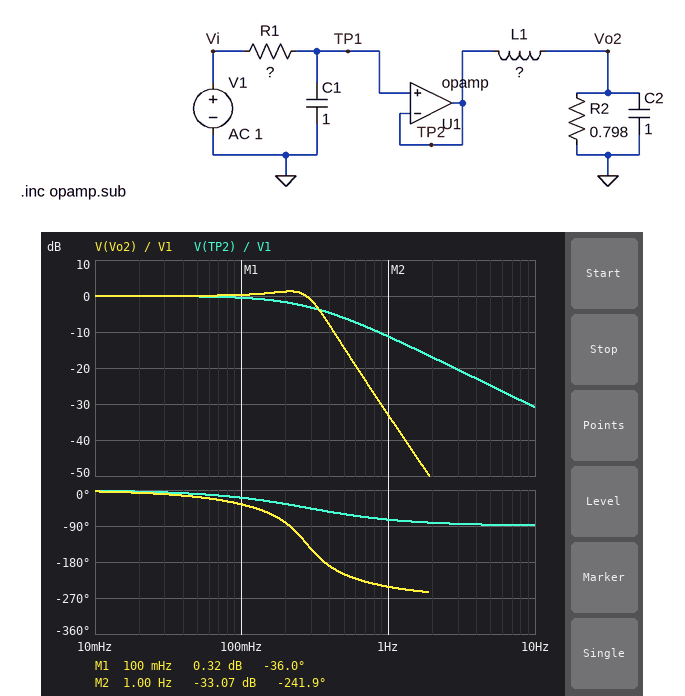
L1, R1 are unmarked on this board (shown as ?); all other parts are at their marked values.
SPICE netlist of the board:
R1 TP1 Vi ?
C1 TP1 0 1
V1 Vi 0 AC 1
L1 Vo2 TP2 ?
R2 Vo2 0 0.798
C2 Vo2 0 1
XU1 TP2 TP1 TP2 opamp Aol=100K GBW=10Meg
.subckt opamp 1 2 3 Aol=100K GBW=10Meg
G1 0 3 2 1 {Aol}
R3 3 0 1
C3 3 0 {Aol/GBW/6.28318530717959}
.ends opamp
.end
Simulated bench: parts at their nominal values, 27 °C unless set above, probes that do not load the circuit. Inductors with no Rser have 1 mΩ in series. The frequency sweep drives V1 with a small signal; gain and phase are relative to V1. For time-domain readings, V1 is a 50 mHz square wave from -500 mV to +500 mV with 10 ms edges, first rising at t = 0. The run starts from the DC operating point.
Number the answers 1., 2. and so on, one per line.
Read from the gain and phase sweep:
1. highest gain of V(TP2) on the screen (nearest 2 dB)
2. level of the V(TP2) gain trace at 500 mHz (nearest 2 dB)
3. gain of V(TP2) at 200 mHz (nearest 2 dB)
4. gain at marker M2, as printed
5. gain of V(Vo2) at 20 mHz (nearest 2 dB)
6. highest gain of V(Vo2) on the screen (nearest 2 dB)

1. 0 dB
2. -6 dB
3. -2 dB
4. -33.07 dB
5. 0 dB
6. 2 dB
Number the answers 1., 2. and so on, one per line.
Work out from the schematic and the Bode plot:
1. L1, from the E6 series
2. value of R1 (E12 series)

1. 330 mH
2. 0.56 Ω
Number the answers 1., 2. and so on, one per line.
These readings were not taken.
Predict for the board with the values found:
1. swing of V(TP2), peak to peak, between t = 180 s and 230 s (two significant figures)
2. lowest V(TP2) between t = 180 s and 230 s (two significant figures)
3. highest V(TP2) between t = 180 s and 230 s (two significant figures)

1. 1.0 V
2. -500 mV
3. 500 mV
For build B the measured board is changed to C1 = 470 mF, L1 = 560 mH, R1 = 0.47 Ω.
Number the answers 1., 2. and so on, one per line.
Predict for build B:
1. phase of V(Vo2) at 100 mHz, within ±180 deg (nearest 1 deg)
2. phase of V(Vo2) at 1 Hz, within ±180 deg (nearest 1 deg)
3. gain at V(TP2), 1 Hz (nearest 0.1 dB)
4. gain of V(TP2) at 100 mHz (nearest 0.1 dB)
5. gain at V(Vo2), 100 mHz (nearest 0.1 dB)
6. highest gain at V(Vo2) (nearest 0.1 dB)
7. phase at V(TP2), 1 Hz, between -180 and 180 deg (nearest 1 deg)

1. -37 deg
2. 138 deg
3. -4.7 dB
4. -0.1 dB
5. 0.9 dB
6. 1.4 dB
7. -54 deg
